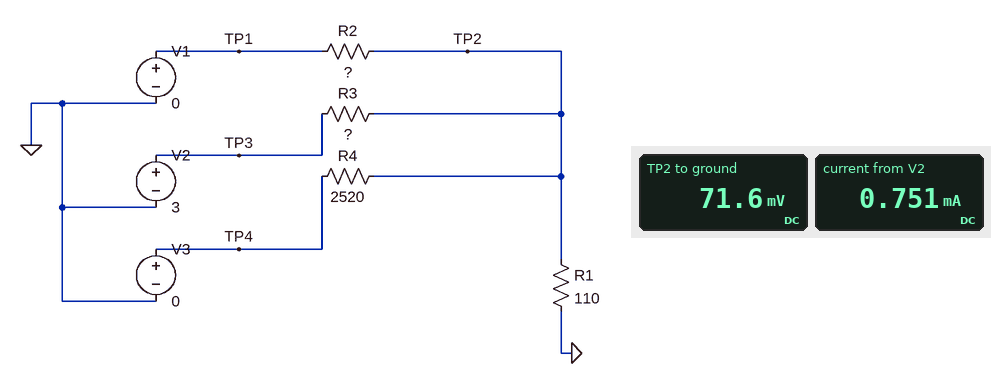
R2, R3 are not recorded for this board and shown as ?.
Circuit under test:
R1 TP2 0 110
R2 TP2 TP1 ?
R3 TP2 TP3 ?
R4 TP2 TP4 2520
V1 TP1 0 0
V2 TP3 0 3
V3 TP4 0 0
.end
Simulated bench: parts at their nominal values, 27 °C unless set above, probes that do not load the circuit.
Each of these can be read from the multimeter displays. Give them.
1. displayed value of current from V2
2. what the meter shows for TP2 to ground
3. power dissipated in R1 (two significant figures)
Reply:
0.751 mA
71.6 mV
47 µW
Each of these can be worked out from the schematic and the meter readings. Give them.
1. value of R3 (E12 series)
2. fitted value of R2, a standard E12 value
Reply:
3.9 kΩ
1 kΩ
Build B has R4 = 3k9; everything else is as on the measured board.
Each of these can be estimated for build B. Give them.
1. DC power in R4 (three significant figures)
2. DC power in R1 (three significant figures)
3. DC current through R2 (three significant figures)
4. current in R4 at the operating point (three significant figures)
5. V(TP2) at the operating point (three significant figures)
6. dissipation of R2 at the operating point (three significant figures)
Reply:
1.35 µW
47.8 µW
72.5 µA
18.6 µA
72.5 mV
5.26 µW
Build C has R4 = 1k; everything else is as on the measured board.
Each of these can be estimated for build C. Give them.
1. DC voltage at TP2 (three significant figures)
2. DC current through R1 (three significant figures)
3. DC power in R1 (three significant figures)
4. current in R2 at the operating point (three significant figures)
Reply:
67.8 mV
616 µA
41.8 µW
67.8 µA
